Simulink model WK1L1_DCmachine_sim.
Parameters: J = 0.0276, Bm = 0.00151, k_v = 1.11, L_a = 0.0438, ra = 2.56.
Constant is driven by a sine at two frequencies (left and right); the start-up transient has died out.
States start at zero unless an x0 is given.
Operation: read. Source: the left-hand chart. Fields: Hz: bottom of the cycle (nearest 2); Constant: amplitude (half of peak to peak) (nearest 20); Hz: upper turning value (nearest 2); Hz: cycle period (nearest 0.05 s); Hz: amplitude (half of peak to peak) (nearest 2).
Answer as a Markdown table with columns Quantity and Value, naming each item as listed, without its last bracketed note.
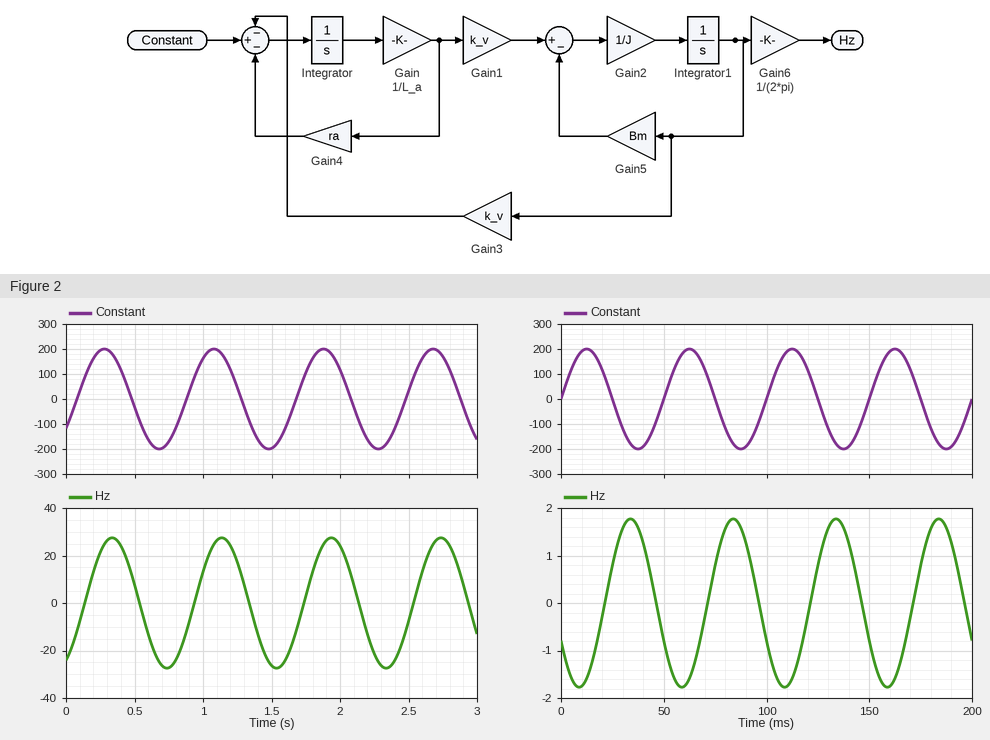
| Quantity | Value |
|---|---|
| Hz: bottom of the cycle | -28 |
| Constant: amplitude (half of peak to peak) | 200 |
| Hz: upper turning value | 28 |
| Hz: cycle period | 0.80 s |
| Hz: amplitude (half of peak to peak) | 28 |
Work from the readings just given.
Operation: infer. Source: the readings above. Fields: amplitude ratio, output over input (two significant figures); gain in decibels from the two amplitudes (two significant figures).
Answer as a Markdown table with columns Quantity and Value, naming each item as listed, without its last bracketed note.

| Quantity | Value |
|---|---|
| amplitude ratio, output over input | 0.14 |
| gain in decibels from the two amplitudes | -17 dB |
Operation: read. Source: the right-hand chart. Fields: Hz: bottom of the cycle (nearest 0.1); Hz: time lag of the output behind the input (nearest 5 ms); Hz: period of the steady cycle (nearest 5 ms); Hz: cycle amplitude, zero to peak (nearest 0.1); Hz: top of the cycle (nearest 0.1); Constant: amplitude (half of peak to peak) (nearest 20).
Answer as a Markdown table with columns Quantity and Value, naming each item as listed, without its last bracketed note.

| Quantity | Value |
|---|---|
| Hz: bottom of the cycle | -1.8 |
| Hz: time lag of the output behind the input | 20 ms |
| Hz: period of the steady cycle | 50 ms |
| Hz: cycle amplitude, zero to peak | 1.8 |
| Hz: top of the cycle | 1.8 |
| Constant: amplitude (half of peak to peak) | 200 |
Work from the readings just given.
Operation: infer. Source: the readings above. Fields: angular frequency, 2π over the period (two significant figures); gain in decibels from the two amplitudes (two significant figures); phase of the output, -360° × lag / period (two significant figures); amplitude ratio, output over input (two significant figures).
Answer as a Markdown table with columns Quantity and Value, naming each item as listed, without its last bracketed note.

| Quantity | Value |
|---|---|
| angular frequency, 2π over the period | 0.13 rad/ms |
| gain in decibels from the two amplitudes | -41 dB |
| phase of the output, -360° × lag / period | -140° |
| amplitude ratio, output over input | 0.0090 |
